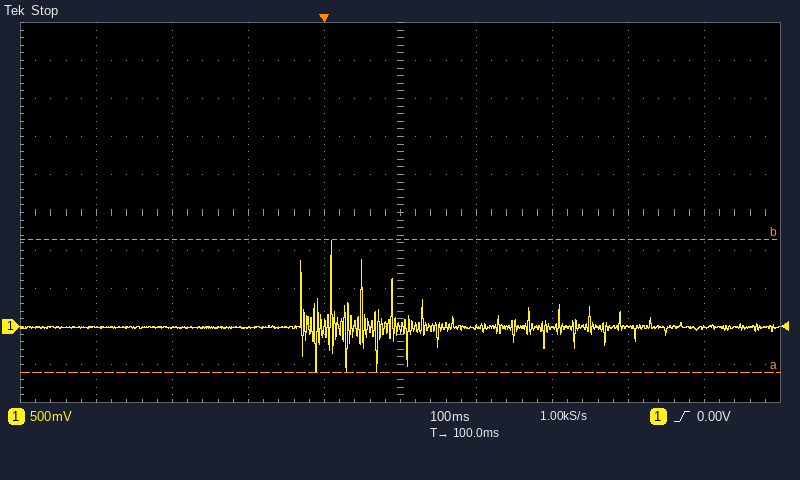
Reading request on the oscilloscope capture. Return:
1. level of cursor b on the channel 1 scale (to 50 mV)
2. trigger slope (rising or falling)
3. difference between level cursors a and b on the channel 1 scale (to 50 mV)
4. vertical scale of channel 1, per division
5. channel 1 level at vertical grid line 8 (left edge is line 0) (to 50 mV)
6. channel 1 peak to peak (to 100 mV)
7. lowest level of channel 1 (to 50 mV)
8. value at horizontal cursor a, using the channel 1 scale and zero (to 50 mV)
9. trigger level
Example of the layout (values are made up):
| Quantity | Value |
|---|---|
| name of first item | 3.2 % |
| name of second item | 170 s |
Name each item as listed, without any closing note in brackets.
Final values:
| Quantity | Value |
|---|---|
| level of cursor b on the channel 1 scale | 1.15 V |
| trigger slope | rising |
| difference between level cursors a and b on the channel 1 scale | 1.75 V |
| vertical scale of channel 1, per division | 500 mV |
| channel 1 level at vertical grid line 8 (left edge is line 0) | 0 mV |
| channel 1 peak to peak | 1.70 V |
| lowest level of channel 1 | -600 mV |
| value at horizontal cursor a, using the channel 1 scale and zero | -600 mV |
| trigger level | 0.00 V |
